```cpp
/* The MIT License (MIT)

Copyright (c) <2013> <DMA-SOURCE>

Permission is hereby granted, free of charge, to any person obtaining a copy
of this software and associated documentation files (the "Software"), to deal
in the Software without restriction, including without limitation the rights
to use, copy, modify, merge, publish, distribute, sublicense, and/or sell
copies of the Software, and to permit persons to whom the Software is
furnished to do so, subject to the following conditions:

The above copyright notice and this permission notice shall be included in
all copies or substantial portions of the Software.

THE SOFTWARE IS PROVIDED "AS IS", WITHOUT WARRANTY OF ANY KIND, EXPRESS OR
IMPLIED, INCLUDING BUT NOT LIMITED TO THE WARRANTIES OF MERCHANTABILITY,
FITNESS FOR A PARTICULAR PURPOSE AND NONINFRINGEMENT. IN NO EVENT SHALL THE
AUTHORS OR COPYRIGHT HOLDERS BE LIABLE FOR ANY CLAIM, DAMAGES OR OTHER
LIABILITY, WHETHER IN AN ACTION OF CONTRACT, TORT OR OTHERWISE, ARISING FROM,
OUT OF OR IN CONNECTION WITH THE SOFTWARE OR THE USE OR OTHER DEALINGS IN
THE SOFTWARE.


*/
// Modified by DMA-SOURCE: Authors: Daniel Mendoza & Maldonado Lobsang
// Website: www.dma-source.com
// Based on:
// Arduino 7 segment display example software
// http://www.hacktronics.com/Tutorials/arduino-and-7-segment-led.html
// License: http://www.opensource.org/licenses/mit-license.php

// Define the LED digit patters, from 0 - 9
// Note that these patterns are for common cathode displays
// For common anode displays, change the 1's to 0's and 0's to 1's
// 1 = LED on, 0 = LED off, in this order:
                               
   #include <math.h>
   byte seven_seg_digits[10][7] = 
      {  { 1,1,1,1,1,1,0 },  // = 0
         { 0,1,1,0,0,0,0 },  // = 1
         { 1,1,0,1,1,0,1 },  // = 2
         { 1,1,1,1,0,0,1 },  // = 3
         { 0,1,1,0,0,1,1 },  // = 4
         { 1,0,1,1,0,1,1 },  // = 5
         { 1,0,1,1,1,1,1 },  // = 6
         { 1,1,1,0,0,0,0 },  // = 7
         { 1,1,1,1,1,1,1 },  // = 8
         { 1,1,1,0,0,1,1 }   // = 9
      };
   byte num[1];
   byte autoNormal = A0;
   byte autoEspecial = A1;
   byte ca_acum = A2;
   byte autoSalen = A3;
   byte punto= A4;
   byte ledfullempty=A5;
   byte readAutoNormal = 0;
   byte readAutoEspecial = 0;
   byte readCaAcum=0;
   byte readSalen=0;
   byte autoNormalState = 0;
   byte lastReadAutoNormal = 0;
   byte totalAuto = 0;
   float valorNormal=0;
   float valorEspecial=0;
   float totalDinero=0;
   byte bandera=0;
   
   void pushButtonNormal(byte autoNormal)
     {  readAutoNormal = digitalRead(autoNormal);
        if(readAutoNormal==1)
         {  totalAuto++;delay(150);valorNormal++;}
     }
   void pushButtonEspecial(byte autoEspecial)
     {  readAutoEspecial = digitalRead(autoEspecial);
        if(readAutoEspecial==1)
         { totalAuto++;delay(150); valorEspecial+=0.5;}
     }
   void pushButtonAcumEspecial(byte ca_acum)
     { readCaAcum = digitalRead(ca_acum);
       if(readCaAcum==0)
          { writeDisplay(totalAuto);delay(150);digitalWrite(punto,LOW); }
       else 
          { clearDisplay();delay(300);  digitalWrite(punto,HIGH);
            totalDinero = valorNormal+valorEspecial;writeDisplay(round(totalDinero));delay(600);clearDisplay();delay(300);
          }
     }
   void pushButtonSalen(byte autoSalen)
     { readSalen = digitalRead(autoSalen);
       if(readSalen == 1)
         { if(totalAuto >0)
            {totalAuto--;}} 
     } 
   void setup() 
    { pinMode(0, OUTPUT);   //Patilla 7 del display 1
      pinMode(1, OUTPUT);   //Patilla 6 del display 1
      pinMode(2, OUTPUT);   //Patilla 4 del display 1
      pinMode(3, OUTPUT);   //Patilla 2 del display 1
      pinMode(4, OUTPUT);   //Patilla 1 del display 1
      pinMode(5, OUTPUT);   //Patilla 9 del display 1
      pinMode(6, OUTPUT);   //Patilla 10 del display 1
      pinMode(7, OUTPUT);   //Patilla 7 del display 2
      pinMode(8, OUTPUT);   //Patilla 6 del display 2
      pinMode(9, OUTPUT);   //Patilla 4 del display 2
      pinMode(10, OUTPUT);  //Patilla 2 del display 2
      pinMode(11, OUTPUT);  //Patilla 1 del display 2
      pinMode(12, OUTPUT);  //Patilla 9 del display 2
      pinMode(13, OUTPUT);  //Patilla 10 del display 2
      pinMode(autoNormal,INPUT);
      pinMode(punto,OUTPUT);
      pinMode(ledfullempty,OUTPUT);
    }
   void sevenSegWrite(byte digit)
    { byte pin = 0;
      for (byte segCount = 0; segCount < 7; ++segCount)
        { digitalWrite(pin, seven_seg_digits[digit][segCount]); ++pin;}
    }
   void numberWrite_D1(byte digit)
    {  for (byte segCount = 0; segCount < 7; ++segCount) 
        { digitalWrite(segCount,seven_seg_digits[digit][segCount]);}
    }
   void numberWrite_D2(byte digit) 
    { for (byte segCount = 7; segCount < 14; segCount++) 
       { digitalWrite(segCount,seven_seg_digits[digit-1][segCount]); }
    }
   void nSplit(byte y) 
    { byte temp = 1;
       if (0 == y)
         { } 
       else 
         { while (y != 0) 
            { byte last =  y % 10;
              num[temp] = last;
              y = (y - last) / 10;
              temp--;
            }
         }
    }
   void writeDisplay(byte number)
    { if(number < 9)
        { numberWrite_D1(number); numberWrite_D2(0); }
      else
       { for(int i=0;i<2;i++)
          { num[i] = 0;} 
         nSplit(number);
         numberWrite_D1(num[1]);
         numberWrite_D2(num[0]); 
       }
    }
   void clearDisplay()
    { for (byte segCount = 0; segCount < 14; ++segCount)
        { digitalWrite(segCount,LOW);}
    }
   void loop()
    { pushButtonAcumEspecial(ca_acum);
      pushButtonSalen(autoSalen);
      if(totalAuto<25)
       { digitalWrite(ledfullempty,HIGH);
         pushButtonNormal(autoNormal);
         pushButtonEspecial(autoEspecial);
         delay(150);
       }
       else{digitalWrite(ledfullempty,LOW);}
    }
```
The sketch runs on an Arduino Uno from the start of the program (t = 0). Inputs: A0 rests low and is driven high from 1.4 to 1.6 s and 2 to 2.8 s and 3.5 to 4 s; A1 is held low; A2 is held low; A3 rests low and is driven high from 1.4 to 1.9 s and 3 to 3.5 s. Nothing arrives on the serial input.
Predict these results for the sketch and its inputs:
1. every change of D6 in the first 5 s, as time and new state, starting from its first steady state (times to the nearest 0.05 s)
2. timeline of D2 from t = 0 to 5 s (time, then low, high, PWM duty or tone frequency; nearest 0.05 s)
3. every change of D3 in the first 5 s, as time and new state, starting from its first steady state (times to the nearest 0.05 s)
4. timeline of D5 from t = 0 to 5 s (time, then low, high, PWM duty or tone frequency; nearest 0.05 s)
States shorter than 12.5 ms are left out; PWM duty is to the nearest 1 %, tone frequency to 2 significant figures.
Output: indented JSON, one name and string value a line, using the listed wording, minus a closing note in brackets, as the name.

{
  "every change of D6 in the first 5 s, as time and new state, starting from its first steady state": "0 s low; 3 s high; 3.3 s low",
  "timeline of D2 from t = 0 to 5 s": "0 s high; 3 s low; 3.3 s high",
  "every change of D3 in the first 5 s, as time and new state, starting from its first steady state": "0 s high; 2.55 s low; 3 s high; 3.3 s low; 3.6 s high; 4.05 s low",
  "timeline of D5 from t = 0 to 5 s": "0 s high; 2.55 s low; 3.6 s high; 4.05 s low"
}
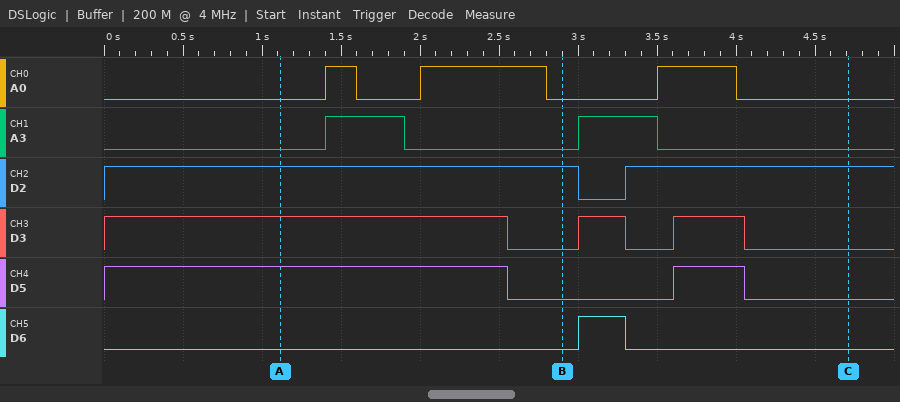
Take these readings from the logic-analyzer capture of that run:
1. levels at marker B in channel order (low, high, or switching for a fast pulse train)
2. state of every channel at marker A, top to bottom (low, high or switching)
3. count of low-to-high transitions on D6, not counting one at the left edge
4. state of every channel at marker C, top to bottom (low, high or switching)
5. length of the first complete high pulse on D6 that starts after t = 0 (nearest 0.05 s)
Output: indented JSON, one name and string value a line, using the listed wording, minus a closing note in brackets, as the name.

{
  "levels at marker B in channel order": "A0 low, A3 low, D2 high, D3 low, D5 low, D6 low",
  "state of every channel at marker A, top to bottom": "A0 low, A3 low, D2 high, D3 high, D5 high, D6 low",
  "count of low-to-high transitions on D6, not counting one at the left edge": "1",
  "state of every channel at marker C, top to bottom": "A0 low, A3 low, D2 high, D3 low, D5 low, D6 low",
  "length of the first complete high pulse on D6 that starts after t = 0": "0.30 s"
}
